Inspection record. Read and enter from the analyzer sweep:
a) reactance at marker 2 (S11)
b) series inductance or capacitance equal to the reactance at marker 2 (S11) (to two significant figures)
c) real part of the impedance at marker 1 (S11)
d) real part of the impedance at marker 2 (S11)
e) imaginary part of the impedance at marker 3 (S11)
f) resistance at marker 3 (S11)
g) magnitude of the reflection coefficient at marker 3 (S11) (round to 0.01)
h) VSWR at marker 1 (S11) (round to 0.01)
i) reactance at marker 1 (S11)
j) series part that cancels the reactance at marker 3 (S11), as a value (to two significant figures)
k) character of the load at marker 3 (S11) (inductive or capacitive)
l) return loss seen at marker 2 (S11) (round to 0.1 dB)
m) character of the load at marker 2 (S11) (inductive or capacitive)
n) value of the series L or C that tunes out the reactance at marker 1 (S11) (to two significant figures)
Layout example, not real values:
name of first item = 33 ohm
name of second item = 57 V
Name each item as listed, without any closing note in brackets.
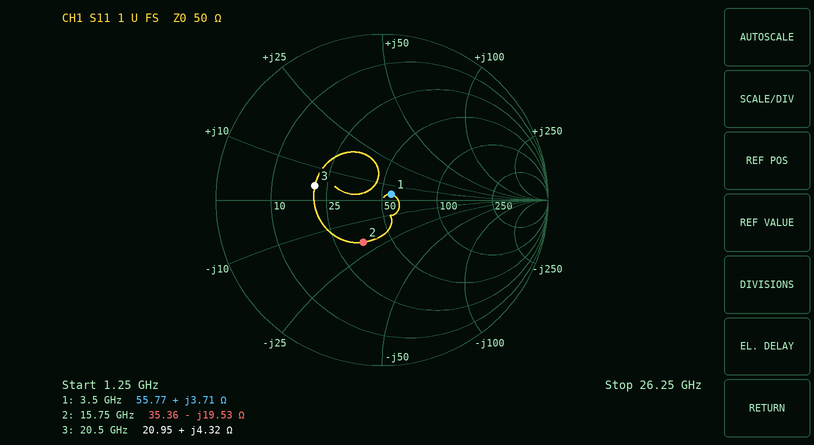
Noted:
reactance at marker 2 = -19.53 Ω
series inductance or capacitance equal to the reactance at marker 2 (S11) = 520 fF
real part of the impedance at marker 1 = 55.77 Ω
real part of the impedance at marker 2 = 35.36 Ω
imaginary part of the impedance at marker 3 = +4.32 Ω
resistance at marker 3 = 20.95 Ω
magnitude of the reflection coefficient at marker 3 (S11) = 0.41
VSWR at marker 1 (S11) = 1.14
reactance at marker 1 = +3.71 Ω
series part that cancels the reactance at marker 3 (S11), as a value = 1.8 pF
character of the load at marker 3 (S11) = inductive
return loss seen at marker 2 (S11) = 11.1 dB
character of the load at marker 2 (S11) = capacitive
value of the series L or C that tunes out the reactance at marker 1 (S11) = 12 pF
